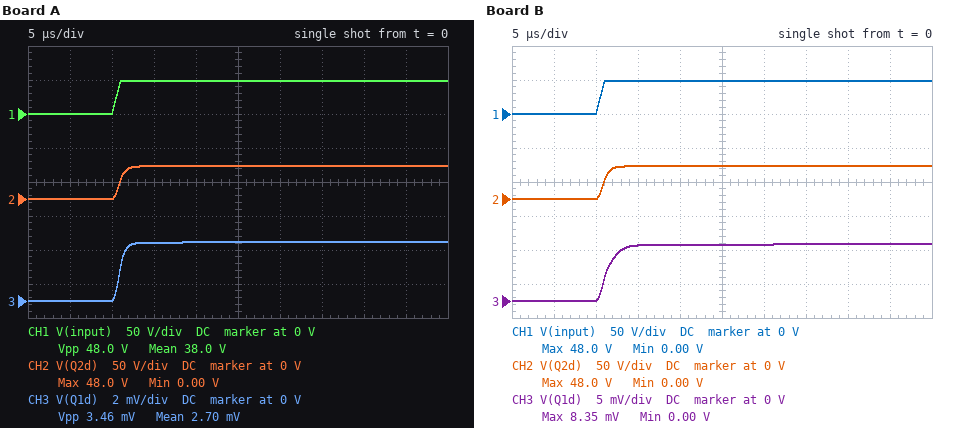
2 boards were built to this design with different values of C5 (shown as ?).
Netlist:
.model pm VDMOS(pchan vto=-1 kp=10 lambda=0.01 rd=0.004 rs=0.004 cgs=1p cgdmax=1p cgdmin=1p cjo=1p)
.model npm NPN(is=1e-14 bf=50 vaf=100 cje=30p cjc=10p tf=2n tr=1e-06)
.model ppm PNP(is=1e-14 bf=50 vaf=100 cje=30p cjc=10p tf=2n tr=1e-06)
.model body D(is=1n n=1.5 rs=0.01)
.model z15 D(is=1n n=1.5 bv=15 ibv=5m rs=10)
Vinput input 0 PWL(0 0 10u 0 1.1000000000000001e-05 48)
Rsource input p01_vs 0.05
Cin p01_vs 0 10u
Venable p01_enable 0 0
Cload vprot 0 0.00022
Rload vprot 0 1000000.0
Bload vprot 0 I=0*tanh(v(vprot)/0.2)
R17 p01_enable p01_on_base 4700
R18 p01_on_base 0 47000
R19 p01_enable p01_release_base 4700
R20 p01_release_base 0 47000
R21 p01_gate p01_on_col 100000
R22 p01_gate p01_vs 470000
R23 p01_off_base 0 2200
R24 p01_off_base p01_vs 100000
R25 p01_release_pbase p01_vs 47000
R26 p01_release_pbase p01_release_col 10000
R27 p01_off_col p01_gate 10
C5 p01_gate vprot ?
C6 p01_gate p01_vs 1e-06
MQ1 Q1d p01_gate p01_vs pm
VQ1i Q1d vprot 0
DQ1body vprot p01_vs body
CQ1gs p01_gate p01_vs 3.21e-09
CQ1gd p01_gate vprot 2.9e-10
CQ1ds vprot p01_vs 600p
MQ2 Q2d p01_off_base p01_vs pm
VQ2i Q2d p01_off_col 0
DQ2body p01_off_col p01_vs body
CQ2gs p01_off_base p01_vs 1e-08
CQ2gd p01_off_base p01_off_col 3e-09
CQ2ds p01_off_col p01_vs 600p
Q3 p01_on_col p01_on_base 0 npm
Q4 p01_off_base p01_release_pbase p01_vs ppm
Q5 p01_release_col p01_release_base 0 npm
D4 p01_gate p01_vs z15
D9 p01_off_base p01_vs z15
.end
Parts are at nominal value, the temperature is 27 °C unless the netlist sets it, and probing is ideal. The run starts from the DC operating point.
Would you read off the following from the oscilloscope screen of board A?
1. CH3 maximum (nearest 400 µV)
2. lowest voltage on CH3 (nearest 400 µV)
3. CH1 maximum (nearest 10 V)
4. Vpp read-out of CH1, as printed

3.6 mV
0 V
50 V
48.0 V
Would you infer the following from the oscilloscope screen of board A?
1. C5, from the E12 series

15 nF
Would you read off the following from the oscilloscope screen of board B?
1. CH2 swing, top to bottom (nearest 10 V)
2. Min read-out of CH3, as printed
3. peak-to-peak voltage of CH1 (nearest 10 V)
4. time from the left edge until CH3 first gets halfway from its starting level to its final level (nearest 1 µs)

50 V
0.00 V
50 V
11 µs
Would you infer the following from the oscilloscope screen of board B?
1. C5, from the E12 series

27 nF
